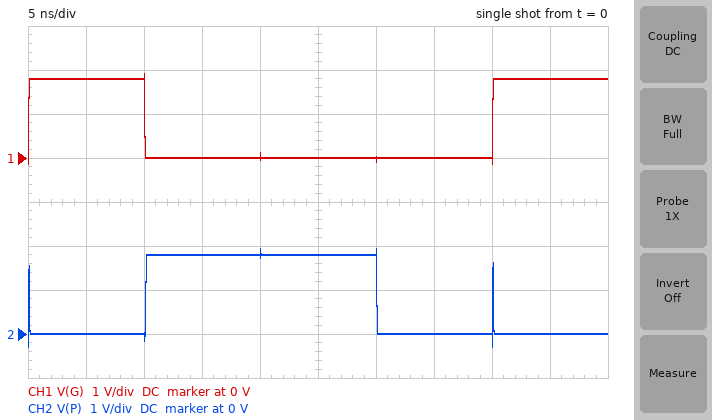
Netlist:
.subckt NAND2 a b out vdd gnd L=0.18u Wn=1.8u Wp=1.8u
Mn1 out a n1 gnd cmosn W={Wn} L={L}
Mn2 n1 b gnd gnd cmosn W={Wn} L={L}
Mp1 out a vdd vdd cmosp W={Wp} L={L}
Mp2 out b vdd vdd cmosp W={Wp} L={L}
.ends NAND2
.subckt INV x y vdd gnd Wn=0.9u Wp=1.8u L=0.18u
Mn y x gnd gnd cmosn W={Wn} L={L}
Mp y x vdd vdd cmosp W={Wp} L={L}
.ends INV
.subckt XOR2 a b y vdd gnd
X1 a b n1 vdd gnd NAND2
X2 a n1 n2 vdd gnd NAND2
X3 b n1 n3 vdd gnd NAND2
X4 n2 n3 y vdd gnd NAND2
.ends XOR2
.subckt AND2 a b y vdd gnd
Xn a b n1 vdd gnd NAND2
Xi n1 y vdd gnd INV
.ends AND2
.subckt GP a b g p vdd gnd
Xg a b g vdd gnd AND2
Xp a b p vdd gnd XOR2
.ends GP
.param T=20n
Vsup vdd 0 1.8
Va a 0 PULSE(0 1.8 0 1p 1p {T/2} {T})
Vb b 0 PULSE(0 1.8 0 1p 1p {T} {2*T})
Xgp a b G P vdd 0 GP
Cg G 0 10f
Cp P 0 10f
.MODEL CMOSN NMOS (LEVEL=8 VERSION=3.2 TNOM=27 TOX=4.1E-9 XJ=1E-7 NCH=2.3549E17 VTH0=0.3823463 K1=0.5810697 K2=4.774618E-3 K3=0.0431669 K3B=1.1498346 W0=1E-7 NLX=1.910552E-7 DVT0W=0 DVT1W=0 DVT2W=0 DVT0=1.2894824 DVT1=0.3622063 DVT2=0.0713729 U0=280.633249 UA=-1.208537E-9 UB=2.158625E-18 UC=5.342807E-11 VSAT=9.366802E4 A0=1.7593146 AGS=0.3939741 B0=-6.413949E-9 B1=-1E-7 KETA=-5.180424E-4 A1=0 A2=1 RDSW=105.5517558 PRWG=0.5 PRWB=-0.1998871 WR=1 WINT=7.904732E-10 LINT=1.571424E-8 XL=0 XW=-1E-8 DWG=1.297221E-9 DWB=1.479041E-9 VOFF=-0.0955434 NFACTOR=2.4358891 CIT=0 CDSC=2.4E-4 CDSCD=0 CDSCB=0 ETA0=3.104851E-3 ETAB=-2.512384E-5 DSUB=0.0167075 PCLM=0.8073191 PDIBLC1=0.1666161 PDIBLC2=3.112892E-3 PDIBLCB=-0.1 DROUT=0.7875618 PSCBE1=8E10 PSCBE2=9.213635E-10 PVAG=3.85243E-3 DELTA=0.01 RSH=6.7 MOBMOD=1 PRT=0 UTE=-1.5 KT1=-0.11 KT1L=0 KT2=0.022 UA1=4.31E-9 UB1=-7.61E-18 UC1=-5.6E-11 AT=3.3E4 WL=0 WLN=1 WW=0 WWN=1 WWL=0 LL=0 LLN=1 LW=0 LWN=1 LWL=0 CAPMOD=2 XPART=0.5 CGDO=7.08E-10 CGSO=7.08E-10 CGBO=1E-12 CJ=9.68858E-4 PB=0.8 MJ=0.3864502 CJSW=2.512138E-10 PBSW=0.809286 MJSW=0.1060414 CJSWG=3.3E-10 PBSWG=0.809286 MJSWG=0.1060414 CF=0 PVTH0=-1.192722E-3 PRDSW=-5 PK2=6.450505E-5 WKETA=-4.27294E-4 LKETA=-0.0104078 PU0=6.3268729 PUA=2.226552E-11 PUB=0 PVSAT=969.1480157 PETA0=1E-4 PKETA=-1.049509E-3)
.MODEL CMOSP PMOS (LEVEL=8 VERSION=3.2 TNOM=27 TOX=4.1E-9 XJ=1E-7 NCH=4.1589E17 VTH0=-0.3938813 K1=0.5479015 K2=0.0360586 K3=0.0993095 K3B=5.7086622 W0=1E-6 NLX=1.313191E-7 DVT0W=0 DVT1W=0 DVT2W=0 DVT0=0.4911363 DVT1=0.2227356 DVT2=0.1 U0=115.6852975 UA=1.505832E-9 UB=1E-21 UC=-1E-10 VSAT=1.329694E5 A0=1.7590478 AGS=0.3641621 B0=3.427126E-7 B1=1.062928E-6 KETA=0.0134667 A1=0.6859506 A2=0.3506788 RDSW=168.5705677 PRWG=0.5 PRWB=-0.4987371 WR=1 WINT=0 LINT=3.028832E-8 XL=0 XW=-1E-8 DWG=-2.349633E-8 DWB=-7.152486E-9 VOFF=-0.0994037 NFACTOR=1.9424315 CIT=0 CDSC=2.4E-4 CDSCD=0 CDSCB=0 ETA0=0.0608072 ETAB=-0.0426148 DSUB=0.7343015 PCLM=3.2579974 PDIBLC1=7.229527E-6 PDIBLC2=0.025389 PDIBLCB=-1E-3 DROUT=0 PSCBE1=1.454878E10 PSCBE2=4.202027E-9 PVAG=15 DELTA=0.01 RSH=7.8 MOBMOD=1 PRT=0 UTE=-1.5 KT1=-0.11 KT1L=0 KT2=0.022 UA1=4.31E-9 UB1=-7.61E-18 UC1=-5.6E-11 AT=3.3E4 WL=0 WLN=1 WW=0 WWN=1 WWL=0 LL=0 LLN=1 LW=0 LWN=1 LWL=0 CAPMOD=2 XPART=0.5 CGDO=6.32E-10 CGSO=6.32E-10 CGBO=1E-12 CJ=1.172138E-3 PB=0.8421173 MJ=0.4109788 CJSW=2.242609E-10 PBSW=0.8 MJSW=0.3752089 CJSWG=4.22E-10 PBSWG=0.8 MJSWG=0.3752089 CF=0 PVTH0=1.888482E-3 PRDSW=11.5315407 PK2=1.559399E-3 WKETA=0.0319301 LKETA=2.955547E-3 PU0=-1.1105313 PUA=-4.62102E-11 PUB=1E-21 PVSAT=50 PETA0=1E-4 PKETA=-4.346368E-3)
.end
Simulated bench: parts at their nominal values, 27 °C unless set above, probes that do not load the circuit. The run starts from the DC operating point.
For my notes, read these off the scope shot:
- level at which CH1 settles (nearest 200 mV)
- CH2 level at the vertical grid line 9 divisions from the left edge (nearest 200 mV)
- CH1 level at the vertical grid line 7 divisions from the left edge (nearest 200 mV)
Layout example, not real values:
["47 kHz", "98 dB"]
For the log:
["1.8 V", "0 V", "0 V"]
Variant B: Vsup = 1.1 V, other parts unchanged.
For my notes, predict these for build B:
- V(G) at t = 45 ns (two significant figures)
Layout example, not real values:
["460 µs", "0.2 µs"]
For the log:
["1.1 V"]
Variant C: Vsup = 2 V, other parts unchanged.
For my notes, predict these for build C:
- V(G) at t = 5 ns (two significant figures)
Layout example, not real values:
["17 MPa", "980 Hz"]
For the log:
["2.0 V"]
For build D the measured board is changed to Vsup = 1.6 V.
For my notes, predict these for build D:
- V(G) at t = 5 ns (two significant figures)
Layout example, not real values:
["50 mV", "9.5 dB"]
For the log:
["1.6 V"]
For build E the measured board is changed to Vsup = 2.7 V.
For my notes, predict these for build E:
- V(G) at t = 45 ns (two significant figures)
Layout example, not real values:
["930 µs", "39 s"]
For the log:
["2.7 V"]
